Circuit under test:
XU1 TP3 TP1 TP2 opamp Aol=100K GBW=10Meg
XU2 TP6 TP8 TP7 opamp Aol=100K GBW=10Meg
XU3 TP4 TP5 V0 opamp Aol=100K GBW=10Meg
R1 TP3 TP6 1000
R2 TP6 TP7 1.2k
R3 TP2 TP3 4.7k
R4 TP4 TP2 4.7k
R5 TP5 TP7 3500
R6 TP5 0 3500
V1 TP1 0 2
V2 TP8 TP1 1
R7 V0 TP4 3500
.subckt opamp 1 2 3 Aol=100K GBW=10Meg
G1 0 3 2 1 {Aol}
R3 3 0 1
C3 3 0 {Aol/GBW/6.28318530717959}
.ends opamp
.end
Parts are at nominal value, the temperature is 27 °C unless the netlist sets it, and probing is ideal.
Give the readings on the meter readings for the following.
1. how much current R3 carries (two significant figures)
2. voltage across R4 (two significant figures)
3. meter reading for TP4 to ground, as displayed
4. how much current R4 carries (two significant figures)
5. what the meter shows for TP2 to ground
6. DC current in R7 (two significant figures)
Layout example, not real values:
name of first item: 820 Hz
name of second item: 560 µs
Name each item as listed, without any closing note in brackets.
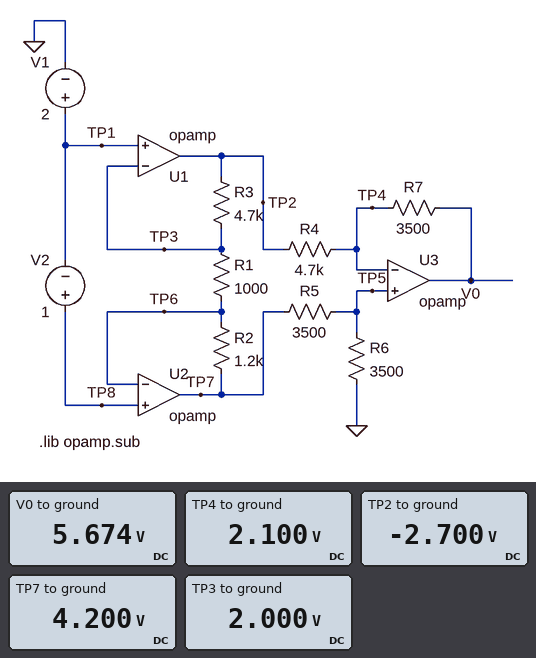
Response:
how much current R3 carries: 1.0 mA
voltage across R4: 4.8 V
meter reading for TP4 to ground, as displayed: 2.100 V
how much current R4 carries: 1.0 mA
what the meter shows for TP2 to ground: -2.700 V
DC current in R7: 1.0 mA
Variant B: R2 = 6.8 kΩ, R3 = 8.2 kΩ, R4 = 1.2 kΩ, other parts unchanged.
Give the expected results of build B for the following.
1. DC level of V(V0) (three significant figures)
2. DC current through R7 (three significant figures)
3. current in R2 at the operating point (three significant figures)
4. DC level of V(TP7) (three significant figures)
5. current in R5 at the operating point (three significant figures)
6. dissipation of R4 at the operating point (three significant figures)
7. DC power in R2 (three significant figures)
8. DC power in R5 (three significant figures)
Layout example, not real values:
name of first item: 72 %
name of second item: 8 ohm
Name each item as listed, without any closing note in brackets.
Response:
DC level of V(V0): 37.3 V
DC current through R7: 9.25 mA
current in R2 at the operating point: 1.00 mA
DC level of V(TP7): 9.80 V
current in R5 at the operating point: 1.40 mA
dissipation of R4 at the operating point: 103 mW
DC power in R2: 6.80 mW
DC power in R5: 6.86 mW
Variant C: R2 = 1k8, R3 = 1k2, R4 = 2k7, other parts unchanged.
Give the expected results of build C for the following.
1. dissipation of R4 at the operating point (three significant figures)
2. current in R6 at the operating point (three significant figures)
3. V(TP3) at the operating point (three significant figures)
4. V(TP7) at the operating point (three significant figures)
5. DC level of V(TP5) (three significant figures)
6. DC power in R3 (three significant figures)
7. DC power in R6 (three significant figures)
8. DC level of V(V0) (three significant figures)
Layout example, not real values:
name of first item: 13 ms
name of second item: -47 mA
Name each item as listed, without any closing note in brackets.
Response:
dissipation of R4 at the operating point: 948 µW
current in R6 at the operating point: 686 µA
V(TP3) at the operating point: 2.00 V
V(TP7) at the operating point: 4.80 V
DC level of V(TP5): 2.40 V
DC power in R3: 1.20 mW
DC power in R6: 1.65 mW
DC level of V(V0): 4.47 V
